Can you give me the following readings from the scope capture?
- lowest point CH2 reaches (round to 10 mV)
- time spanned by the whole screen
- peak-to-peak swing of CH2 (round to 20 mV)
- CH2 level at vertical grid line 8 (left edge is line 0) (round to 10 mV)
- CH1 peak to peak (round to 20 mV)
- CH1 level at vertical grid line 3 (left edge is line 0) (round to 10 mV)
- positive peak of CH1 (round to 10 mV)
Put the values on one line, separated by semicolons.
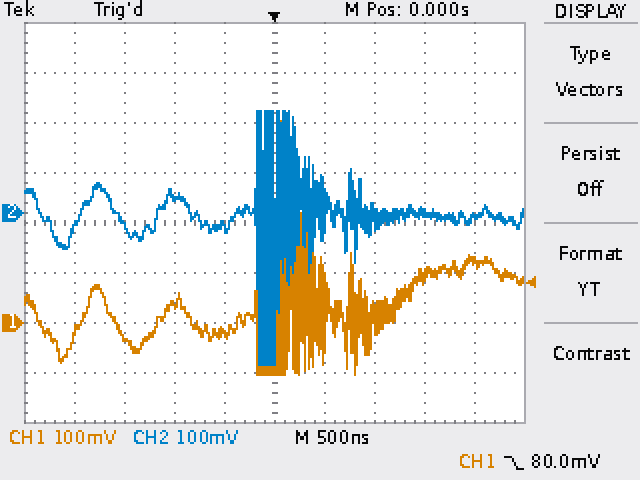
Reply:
-300 mV; 5 µs; 500 mV; 0 mV; 500 mV; 40 mV; 400 mV
